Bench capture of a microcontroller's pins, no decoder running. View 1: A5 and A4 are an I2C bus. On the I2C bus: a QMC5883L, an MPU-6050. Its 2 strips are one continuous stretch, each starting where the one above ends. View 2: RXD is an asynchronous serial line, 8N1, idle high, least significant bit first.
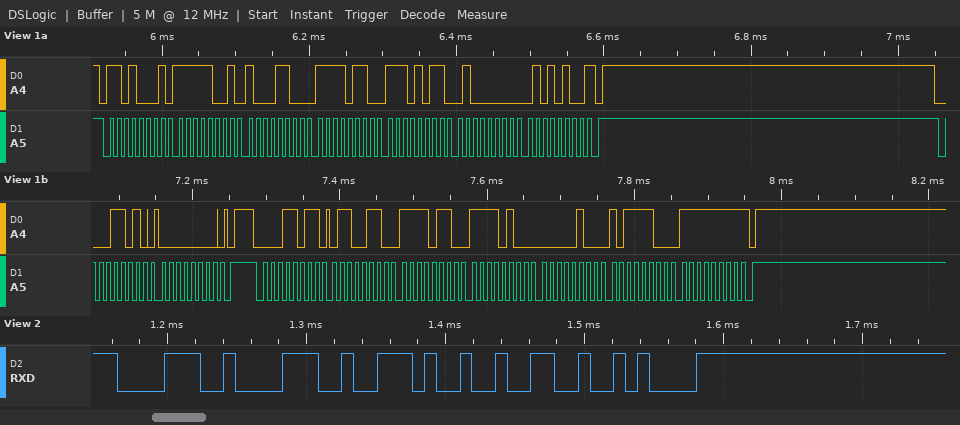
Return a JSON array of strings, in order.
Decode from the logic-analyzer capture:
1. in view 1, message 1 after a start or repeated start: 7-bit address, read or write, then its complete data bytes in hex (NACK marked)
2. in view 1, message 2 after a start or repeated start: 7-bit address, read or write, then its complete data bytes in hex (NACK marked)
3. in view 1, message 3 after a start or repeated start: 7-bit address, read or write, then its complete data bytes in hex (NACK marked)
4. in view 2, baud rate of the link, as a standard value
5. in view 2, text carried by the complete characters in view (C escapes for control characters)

["0x68 read: F9 8C F6 EB 40 54 NACK", "0x0D write: 00", "0x0D read: 66 F6 F4 04 BC FF NACK", "115200 baud", "\"88.2\\n\""]
